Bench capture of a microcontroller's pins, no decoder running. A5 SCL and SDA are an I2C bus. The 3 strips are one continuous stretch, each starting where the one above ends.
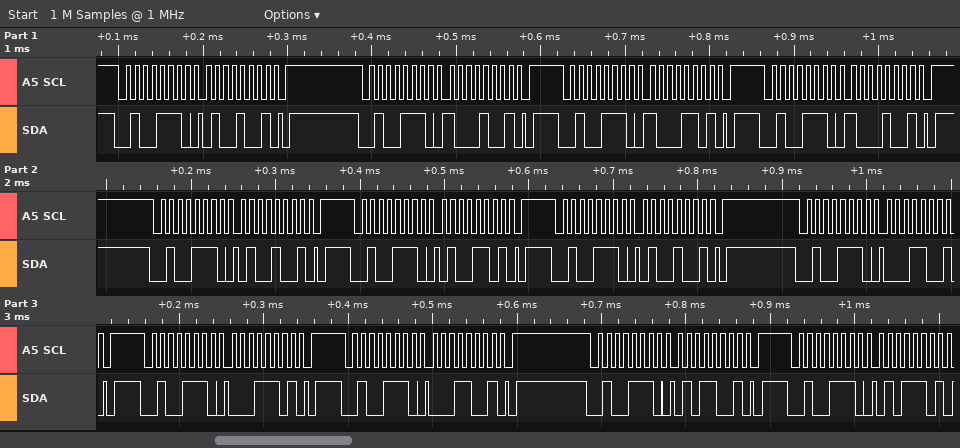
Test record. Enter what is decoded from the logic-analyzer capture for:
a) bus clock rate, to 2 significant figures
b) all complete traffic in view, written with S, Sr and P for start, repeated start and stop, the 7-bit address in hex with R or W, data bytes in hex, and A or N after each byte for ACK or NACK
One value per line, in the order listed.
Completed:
100 kHz
S 27W A 49 A P S 27W A 89 A P S 27W A 8D A P S 27W A 89 A P S 27W A 49 A P S 27W A 4D A P S 27W A 49 A P S 27W A 19 A P S 27W A 1D A P S 27W A 19 A P S 27W A 59 A P S 27W A 5D A
